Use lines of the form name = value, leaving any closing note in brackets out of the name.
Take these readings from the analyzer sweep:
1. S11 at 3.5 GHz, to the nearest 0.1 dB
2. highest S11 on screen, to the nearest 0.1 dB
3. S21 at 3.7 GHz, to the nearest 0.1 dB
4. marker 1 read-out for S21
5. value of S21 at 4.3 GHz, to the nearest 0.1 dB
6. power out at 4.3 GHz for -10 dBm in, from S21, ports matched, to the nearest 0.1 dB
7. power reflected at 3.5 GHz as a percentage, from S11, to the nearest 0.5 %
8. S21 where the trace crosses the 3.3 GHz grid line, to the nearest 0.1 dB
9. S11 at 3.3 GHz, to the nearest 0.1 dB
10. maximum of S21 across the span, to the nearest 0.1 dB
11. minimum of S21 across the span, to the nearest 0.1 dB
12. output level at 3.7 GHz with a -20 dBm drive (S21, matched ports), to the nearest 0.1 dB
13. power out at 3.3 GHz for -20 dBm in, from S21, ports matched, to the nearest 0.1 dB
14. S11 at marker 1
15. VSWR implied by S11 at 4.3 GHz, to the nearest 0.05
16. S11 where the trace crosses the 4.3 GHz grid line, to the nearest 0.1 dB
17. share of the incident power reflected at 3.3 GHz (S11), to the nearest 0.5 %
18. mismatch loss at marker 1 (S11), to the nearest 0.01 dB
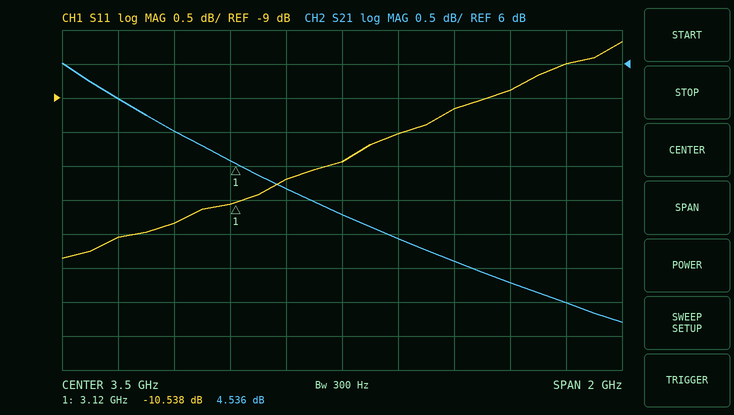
S11 at 3.5 GHz, to the nearest 0.1 dB = -9.9 dB
highest S11 on screen, to the nearest 0.1 dB = -8.2 dB
S21 at 3.7 GHz, to the nearest 0.1 dB = 3.4 dB
marker 1 read-out for S21 = 4.536 dB
value of S21 at 4.3 GHz, to the nearest 0.1 dB = 2.5 dB
power out at 4.3 GHz for -10 dBm in, from S21, ports matched, to the nearest 0.1 dB = -7.5 dBm
power reflected at 3.5 GHz as a percentage, from S11, to the nearest 0.5 % = 10.0 %
S21 where the trace crosses the 3.3 GHz grid line, to the nearest 0.1 dB = 4.2 dB
S11 at 3.3 GHz, to the nearest 0.1 dB = -10.2 dB
maximum of S21 across the span, to the nearest 0.1 dB = 6.0 dB
minimum of S21 across the span, to the nearest 0.1 dB = 2.2 dB
output level at 3.7 GHz with a -20 dBm drive (S21, matched ports), to the nearest 0.1 dB = -16.6 dBm
power out at 3.3 GHz for -20 dBm in, from S21, ports matched, to the nearest 0.1 dB = -15.8 dBm
S11 at marker 1 = -10.538 dB
VSWR implied by S11 at 4.3 GHz, to the nearest 0.05 = 2.20
S11 where the trace crosses the 4.3 GHz grid line, to the nearest 0.1 dB = -8.5 dB
share of the incident power reflected at 3.3 GHz (S11), to the nearest 0.5 % = 9.5 %
mismatch loss at marker 1 (S11), to the nearest 0.01 dB = 0.40 dB
